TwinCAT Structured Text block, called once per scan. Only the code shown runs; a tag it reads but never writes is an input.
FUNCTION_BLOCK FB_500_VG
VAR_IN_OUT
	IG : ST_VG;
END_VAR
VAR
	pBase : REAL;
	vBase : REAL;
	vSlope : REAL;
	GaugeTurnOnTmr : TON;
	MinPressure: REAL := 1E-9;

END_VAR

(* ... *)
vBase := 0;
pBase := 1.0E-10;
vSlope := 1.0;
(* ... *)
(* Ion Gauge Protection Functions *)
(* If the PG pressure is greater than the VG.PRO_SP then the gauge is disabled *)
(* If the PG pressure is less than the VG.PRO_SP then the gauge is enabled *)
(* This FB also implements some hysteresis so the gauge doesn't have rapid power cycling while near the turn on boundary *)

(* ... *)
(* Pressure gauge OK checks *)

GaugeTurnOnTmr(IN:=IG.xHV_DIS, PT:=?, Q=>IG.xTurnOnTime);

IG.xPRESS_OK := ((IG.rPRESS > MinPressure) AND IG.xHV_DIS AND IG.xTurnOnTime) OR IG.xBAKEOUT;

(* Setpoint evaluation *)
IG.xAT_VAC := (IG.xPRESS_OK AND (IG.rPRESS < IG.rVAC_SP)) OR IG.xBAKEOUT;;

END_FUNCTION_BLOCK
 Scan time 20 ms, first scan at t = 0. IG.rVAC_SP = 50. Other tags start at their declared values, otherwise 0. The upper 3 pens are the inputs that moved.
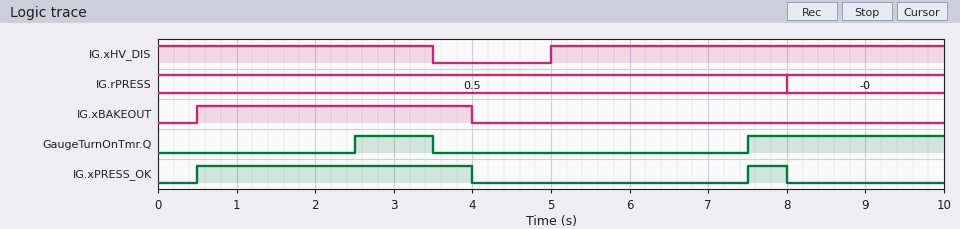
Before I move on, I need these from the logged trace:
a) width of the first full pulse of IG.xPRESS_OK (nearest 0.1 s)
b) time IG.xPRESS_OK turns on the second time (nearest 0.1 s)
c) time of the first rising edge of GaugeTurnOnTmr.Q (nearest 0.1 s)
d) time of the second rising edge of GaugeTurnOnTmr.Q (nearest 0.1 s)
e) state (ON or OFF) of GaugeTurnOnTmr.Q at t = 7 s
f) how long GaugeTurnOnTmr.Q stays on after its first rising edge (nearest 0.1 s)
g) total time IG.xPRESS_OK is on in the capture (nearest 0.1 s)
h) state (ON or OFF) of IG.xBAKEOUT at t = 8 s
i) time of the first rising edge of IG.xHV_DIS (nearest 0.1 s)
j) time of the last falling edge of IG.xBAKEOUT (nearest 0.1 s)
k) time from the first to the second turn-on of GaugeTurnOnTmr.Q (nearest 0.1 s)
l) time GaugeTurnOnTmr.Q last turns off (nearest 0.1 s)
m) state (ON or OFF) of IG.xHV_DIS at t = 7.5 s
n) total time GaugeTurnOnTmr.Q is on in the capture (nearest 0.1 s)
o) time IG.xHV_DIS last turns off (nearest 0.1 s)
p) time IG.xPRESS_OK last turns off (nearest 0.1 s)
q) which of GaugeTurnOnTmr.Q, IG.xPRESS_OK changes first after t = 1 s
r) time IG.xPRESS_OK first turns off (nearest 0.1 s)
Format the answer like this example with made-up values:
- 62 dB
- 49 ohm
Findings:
- 3.5 s
- 7.5 s
- 2.5 s
- 7.5 s
- OFF
- 1.0 s
- 4.0 s
- OFF
- 5.0 s
- 4.0 s
- 5.0 s
- 3.5 s
- ON
- 3.5 s
- 3.5 s
- 8.0 s
- GaugeTurnOnTmr.Q
- 4.0 s
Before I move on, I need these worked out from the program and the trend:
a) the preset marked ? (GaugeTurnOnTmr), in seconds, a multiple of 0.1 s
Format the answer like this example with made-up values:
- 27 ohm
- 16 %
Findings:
- 2.5 s
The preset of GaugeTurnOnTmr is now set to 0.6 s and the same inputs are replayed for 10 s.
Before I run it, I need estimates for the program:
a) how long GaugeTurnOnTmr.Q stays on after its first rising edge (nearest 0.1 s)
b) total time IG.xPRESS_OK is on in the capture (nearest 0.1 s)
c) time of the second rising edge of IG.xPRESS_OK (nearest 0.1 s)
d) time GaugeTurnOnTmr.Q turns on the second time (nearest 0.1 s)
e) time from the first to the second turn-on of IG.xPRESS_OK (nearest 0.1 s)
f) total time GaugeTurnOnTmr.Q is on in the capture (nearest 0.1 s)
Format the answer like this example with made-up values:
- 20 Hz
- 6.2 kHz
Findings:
- 2.9 s
- 5.9 s
- 5.6 s
- 5.6 s
- 5.1 s
- 7.3 s
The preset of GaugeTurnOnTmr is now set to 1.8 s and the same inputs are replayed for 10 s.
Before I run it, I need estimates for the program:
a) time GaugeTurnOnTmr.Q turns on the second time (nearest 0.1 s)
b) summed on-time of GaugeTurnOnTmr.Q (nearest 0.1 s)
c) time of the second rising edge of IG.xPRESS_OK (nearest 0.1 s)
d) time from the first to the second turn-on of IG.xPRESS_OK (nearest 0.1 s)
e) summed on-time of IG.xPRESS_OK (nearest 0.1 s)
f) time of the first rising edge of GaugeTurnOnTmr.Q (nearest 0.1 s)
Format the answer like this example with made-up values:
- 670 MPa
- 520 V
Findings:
- 6.8 s
- 4.9 s
- 6.8 s
- 6.3 s
- 4.7 s
- 1.8 s
